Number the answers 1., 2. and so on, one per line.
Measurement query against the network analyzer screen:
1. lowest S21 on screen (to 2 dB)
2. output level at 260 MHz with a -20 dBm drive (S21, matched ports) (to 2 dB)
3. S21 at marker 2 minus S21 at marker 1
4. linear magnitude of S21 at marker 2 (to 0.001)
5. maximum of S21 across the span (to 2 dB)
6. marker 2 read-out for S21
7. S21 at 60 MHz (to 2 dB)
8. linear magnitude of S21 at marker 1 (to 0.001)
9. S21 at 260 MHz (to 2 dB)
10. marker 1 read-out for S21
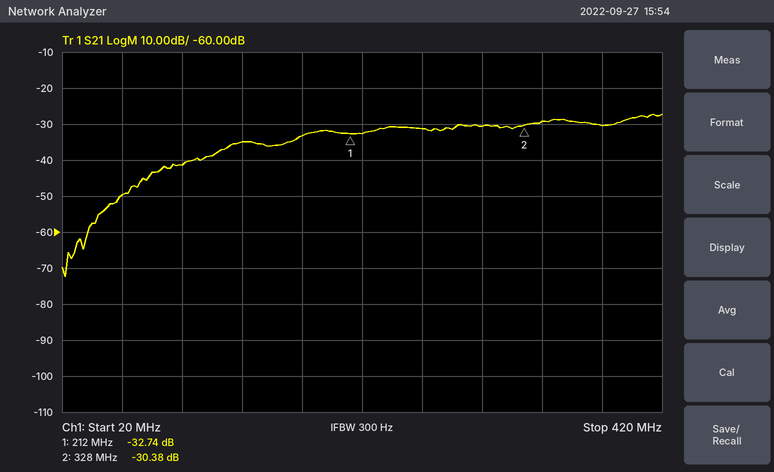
1. -72 dB
2. -52 dBm
3. 2.36 dB
4. 0.030
5. -28 dB
6. -30.38 dB
7. -50 dB
8. 0.023
9. -32 dB
10. -32.74 dB
